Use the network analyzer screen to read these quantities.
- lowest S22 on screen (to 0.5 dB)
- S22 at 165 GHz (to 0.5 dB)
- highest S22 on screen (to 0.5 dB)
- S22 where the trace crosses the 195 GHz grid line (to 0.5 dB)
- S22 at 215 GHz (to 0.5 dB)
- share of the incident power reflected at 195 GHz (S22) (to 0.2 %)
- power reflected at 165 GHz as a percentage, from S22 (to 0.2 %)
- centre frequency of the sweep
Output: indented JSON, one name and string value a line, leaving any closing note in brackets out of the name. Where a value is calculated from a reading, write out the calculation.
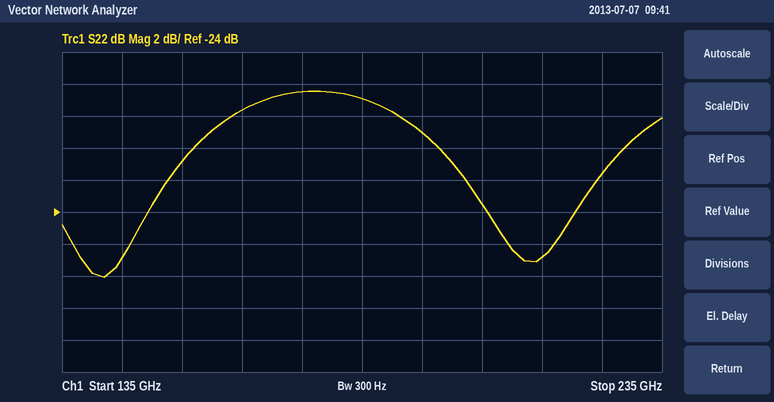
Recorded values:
{
  "lowest S22 on screen": "-28.0 dB",
  "S22 at 165 GHz": "-17.5 dB",
  "highest S22 on screen": "-16.5 dB",
  "S22 where the trace crosses the 195 GHz grid line": "-19.0 dB",
  "S22 at 215 GHz": "-27.0 dB",
  "share of the incident power reflected at 195 GHz (S22)": "10^(-19/10) ≈ 1.26 %, so 1.2 % to the nearest 0.2 %",
  "power reflected at 165 GHz as a percentage, from S22": "10^(-17.5/10) ≈ 1.8 %",
  "centre frequency of the sweep": "185 GHz"
}
